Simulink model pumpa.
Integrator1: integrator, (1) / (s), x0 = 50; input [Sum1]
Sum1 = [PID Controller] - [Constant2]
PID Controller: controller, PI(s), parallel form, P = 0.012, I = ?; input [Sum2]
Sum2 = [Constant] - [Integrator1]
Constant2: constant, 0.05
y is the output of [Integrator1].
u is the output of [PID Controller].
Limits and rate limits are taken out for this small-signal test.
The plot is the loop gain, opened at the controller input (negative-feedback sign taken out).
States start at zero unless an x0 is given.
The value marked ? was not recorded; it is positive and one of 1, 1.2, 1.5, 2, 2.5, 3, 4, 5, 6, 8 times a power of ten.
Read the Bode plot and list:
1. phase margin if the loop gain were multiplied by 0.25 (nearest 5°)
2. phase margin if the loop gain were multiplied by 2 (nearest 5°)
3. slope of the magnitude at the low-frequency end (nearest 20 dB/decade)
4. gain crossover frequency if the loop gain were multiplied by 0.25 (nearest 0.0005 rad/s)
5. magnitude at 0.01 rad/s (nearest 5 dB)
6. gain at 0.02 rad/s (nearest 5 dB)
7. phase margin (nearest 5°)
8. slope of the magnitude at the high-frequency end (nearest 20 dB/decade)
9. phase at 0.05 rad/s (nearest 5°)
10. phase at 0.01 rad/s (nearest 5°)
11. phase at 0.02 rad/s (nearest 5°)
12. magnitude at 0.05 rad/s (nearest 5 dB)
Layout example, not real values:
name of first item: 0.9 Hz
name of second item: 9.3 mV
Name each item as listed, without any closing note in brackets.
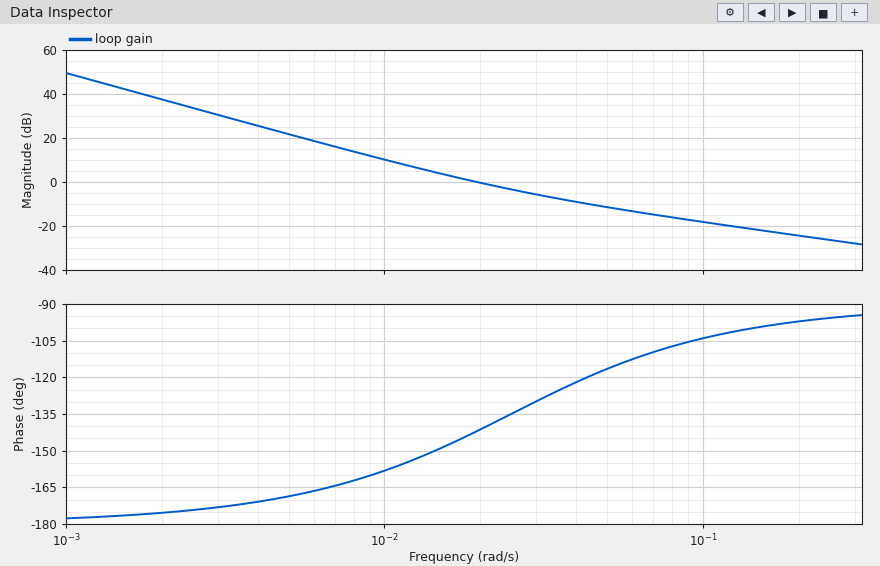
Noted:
phase margin if the loop gain were multiplied by 0.25: 20°
phase margin if the loop gain were multiplied by 2: 50°
slope of the magnitude at the low-frequency end: -40 dB/decade
gain crossover frequency if the loop gain were multiplied by 0.25: 0.0090 rad/s
magnitude at 0.01 rad/s: 10 dB
gain at 0.02 rad/s: 0 dB
phase margin: 40°
slope of the magnitude at the high-frequency end: -20 dB/decade
phase at 0.05 rad/s: -115°
phase at 0.01 rad/s: -160°
phase at 0.02 rad/s: -140°
magnitude at 0.05 rad/s: -10 dB
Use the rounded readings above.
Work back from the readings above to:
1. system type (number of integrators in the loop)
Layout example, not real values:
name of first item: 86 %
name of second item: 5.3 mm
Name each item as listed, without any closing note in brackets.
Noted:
system type: 2
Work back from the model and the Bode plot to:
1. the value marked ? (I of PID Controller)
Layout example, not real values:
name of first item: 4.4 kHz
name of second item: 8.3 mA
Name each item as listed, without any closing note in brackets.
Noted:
the value marked ?: 0.0003
